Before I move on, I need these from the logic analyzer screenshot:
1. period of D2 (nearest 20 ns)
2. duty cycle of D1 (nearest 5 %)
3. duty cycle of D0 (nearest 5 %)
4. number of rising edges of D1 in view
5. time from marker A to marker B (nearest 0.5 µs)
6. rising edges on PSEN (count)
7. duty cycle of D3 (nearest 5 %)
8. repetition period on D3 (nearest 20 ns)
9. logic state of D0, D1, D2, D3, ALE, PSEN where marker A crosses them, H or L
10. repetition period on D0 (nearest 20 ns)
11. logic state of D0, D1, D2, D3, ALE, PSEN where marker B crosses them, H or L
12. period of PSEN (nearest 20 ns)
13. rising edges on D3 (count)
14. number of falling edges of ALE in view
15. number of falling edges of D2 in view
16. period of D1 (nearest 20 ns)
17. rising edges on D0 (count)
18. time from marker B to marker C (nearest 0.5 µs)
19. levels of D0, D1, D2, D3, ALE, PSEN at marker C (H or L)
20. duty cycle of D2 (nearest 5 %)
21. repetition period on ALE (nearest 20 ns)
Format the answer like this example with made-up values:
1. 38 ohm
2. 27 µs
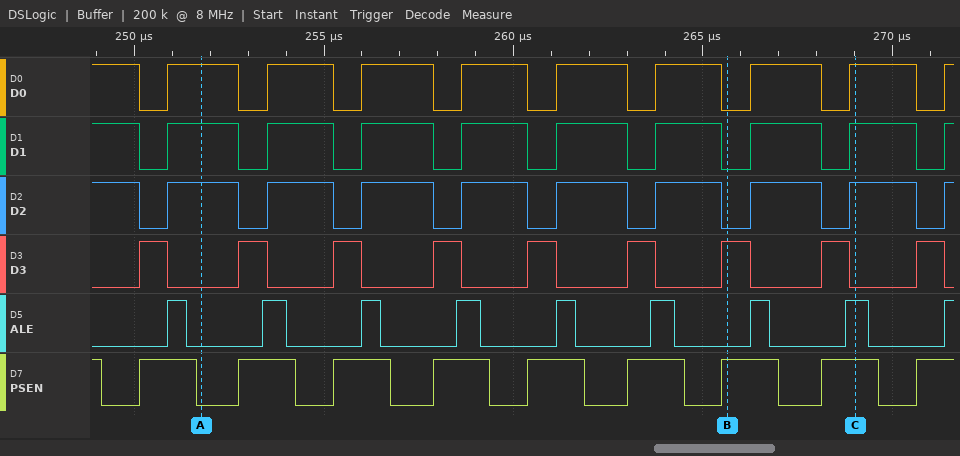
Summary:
1. 2560 ns
2. 70 %
3. 70 %
4. 9
5. 14 µs
6. 9
7. 30 %
8. 2560 ns
9. D0=H, D1=H, D2=H, D3=L, ALE=L, PSEN=L
10. 2560 ns
11. D0=L, D1=L, D2=L, D3=H, ALE=L, PSEN=H
12. 2560 ns
13. 9
14. 8
15. 9
16. 2560 ns
17. 9
18. 3.5 µs
19. D0=H, D1=H, D2=H, D3=L, ALE=H, PSEN=H
20. 70 %
21. 2560 ns
